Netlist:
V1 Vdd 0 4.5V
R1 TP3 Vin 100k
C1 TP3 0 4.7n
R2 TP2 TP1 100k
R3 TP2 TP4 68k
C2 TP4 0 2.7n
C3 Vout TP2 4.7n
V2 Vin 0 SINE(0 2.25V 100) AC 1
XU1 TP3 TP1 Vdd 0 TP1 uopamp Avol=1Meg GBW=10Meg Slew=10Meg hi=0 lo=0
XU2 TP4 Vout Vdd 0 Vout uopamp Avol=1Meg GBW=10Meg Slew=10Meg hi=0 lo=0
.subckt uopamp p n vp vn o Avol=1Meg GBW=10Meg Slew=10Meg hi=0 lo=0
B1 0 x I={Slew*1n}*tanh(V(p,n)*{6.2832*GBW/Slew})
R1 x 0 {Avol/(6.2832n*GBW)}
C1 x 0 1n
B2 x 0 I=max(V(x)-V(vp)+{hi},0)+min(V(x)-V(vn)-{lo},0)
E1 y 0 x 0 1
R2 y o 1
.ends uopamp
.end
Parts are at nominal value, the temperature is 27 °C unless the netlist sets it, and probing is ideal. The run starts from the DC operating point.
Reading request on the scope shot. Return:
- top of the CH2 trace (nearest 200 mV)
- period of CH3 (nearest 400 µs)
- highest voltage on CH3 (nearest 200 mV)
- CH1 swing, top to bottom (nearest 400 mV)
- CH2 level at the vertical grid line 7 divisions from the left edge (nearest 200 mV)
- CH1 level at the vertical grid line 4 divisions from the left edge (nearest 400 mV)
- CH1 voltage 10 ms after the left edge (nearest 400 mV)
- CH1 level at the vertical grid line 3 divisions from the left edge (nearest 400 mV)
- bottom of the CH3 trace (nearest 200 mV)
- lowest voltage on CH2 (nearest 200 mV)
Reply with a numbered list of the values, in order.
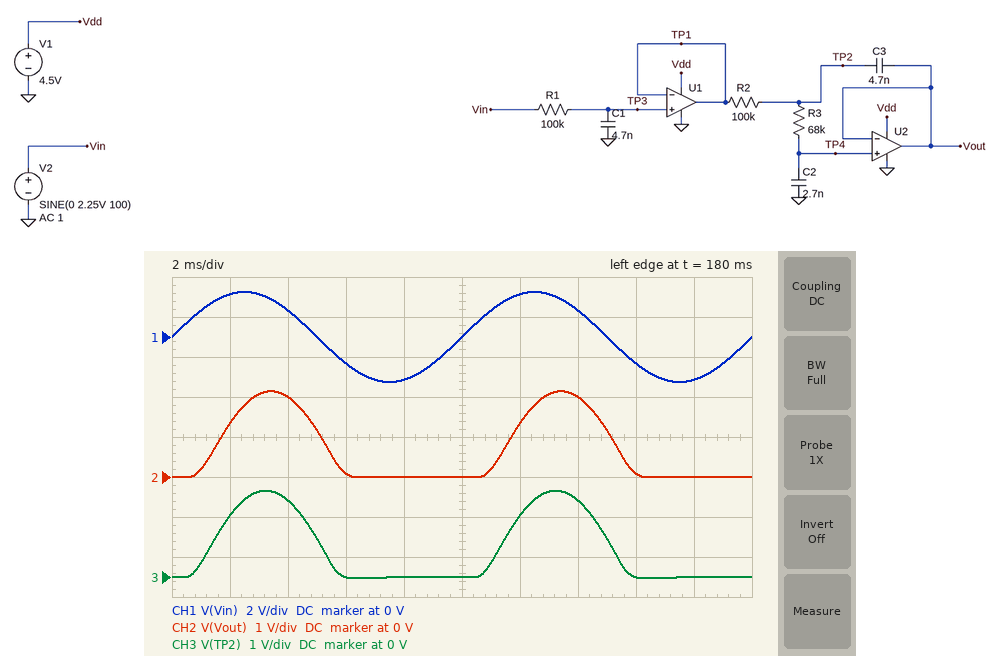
1. 2.2 V
2. 10.0 ms
3. 2.2 V
4. 4.4 V
5. 2.0 V
6. -2.0 V
7. 0 V
8. -1.2 V
9. 0 V
10. 0 V
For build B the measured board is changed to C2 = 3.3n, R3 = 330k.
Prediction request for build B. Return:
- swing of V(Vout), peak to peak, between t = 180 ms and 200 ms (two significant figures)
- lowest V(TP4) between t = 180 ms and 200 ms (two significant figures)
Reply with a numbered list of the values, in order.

1. 1.8 V
2. -3.9 mV
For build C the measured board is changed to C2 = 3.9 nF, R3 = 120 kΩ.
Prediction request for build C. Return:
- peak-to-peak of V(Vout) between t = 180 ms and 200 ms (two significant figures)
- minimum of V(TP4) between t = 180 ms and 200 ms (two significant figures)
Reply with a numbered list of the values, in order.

1. 2.0 V
2. -9.7 mV
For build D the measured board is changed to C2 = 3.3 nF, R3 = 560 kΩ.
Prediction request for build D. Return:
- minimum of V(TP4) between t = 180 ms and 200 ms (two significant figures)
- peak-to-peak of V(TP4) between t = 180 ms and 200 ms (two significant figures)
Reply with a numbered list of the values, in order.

1. 64 mV
2. 1.5 V
